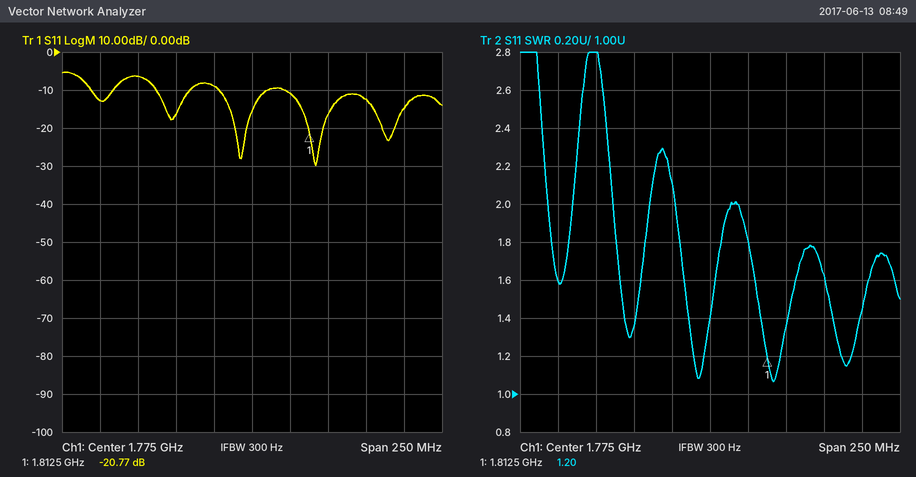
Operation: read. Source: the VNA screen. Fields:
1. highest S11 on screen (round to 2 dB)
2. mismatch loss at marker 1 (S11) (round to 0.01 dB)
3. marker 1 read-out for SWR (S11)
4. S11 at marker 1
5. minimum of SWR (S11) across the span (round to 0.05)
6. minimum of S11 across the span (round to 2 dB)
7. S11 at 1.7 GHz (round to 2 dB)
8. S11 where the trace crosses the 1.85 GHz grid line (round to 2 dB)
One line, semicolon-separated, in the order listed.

-6 dB; 0.04 dB; 1.20; -20.77 dB; 1.05; -30 dB; -6 dB; -12 dB
